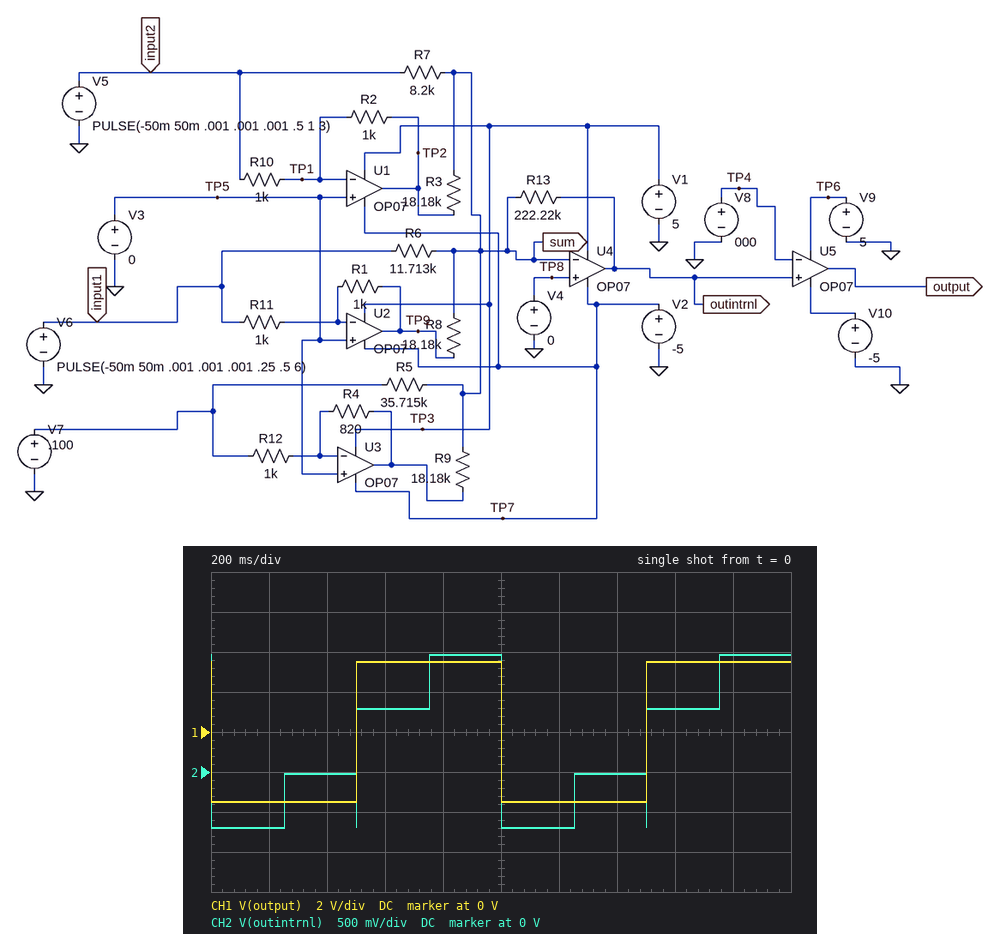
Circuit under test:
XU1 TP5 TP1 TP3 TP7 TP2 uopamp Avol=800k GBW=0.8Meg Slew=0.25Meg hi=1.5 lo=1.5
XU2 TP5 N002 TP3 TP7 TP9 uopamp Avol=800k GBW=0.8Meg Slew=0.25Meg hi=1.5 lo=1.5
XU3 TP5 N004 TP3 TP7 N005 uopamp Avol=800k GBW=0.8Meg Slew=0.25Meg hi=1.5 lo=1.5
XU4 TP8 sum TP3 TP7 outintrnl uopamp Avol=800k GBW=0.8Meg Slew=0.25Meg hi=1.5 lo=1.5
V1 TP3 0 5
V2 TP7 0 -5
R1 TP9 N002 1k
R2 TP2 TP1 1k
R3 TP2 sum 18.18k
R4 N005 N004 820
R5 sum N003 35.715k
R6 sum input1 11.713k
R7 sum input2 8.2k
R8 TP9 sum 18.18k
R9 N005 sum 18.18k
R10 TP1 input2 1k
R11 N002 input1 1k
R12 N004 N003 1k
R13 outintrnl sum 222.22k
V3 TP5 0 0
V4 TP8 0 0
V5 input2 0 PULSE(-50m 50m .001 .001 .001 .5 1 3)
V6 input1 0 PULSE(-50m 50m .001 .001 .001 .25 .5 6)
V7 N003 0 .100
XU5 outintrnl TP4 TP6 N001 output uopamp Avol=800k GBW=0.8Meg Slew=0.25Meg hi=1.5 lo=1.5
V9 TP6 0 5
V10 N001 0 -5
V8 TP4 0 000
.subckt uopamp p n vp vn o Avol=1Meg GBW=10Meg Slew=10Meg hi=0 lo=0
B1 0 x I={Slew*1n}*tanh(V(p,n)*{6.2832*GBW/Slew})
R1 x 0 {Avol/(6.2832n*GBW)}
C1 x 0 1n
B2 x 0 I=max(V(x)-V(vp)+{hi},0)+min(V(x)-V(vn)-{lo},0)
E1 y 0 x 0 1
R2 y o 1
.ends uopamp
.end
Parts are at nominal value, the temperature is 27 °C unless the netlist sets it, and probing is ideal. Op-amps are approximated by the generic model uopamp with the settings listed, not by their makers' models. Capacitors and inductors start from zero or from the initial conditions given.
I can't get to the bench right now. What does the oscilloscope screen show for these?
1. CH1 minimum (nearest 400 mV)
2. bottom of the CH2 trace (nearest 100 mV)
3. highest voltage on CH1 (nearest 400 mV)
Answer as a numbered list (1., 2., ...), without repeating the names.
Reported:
1. -3.6 V
2. -700 mV
3. 3.6 V
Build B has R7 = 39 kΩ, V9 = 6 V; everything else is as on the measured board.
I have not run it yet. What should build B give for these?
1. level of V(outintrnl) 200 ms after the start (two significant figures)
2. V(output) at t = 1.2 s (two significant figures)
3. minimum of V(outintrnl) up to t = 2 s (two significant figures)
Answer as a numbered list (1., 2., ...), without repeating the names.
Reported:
1. 370 mV
2. 4.5 V
3. -280 mV
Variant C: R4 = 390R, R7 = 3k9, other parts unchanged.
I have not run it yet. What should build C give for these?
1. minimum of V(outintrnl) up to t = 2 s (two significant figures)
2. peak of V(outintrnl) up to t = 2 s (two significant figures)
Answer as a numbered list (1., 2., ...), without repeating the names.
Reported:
1. -2.7 V
2. 2.4 V
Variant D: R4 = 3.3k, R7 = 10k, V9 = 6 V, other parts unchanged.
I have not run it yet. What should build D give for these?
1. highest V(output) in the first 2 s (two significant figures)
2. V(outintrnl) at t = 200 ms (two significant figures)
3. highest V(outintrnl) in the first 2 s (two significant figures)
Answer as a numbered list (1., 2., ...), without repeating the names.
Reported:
1. 4.5 V
2. 2.6 V
3. 3.5 V
